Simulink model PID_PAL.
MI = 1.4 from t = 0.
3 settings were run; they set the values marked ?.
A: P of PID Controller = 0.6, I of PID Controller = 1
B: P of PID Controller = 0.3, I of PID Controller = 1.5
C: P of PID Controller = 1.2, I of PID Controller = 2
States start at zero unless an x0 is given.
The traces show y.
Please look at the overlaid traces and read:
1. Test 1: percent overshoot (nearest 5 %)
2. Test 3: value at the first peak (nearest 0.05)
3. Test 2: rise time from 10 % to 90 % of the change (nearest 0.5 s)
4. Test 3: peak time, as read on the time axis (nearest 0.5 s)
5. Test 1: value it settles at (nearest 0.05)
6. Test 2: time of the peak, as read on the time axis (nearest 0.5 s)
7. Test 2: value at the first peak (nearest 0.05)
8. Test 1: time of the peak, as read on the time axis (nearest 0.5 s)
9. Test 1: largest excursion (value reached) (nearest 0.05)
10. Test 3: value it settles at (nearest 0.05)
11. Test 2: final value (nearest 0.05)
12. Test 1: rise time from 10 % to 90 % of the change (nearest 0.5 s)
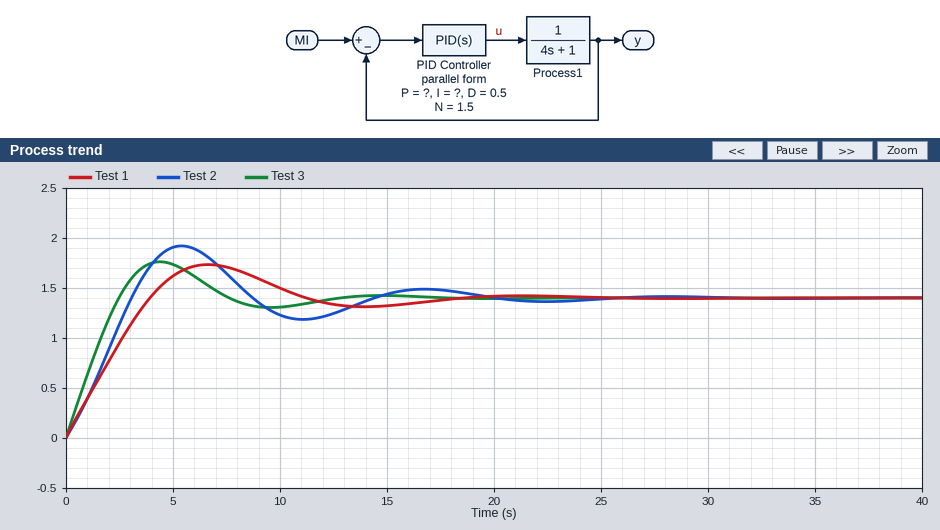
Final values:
25 %
1.75
2.5 s
4.5 s
1.40
5.5 s
1.90
6.5 s
1.75
1.40
1.40
3.0 s
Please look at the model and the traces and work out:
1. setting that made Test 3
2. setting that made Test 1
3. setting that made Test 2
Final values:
C
A
B
